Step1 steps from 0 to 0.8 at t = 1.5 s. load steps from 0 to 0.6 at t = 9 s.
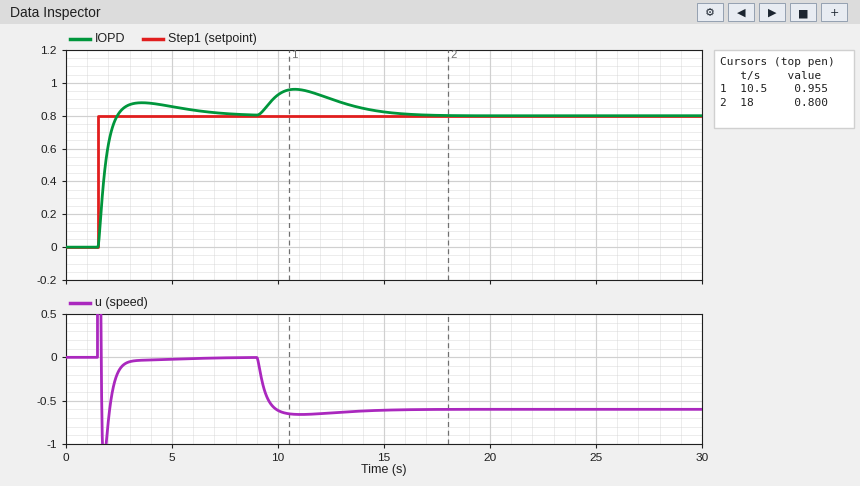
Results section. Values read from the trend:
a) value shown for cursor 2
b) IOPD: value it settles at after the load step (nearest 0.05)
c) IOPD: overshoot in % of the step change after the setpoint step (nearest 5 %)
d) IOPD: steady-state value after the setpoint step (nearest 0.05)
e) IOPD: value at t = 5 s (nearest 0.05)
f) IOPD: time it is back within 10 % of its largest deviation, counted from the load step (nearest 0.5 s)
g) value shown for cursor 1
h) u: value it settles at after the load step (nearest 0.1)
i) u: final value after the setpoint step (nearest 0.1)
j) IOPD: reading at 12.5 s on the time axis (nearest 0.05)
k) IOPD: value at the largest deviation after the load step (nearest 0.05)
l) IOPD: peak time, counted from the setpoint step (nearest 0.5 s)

0.800
0.80
10 %
0.80
0.85
6.5 s
0.955
-0.6
0.0
0.90
0.95
2.0 s
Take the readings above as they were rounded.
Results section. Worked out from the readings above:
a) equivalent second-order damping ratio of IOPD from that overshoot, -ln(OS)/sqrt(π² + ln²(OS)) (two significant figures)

0.59
